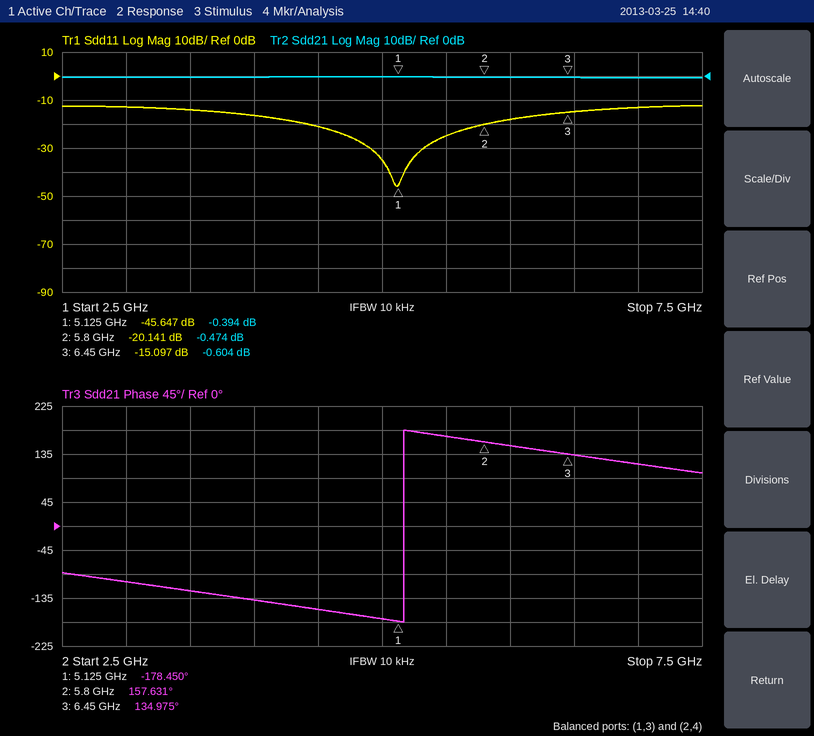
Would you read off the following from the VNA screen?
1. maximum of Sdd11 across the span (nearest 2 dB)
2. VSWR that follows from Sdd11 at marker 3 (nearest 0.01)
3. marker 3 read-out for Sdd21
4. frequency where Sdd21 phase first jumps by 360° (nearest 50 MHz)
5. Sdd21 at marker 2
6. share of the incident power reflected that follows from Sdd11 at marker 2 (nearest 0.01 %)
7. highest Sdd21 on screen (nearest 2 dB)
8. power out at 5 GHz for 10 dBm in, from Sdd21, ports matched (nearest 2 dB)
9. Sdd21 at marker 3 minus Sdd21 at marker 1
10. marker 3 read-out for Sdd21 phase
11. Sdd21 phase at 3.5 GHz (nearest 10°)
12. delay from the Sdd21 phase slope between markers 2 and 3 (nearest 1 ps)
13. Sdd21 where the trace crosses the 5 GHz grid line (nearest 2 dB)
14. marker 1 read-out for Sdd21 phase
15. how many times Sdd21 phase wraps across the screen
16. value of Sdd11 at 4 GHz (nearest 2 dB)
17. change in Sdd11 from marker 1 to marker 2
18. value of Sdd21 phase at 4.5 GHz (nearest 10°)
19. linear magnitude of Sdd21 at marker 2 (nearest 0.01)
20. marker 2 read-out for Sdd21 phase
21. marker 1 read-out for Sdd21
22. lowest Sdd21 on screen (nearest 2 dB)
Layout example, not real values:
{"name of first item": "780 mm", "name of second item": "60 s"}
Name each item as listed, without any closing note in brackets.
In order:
{"maximum of Sdd11 across the span": "-12 dB", "VSWR that follows from Sdd11 at marker 3": "1.43", "marker 3 read-out for Sdd21": "-0.604 dB", "frequency where Sdd21 phase first jumps by 360°": "5.15 GHz", "Sdd21 at marker 2": "-0.474 dB", "share of the incident power reflected that follows from Sdd11 at marker 2": "0.97 %", "highest Sdd21 on screen": "0 dB", "power out at 5 GHz for 10 dBm in, from Sdd21, ports matched": "10 dBm", "Sdd21 at marker 3 minus Sdd21 at marker 1": "-0.210 dB", "marker 3 read-out for Sdd21 phase": "134.975°", "Sdd21 phase at 3.5 GHz": "-120°", "delay from the Sdd21 phase slope between markers 2 and 3": "97 ps", "Sdd21 where the trace crosses the 5 GHz grid line": "0 dB", "marker 1 read-out for Sdd21 phase": "-178.450°", "how many times Sdd21 phase wraps across the screen": "1", "value of Sdd11 at 4 GHz": "-16 dB", "change in Sdd11 from marker 1 to marker 2": "25.506 dB", "value of Sdd21 phase at 4.5 GHz": "-160°", "linear magnitude of Sdd21 at marker 2": "0.95", "marker 2 read-out for Sdd21 phase": "157.631°", "marker 1 read-out for Sdd21": "-0.394 dB", "lowest Sdd21 on screen": "0 dB"}
